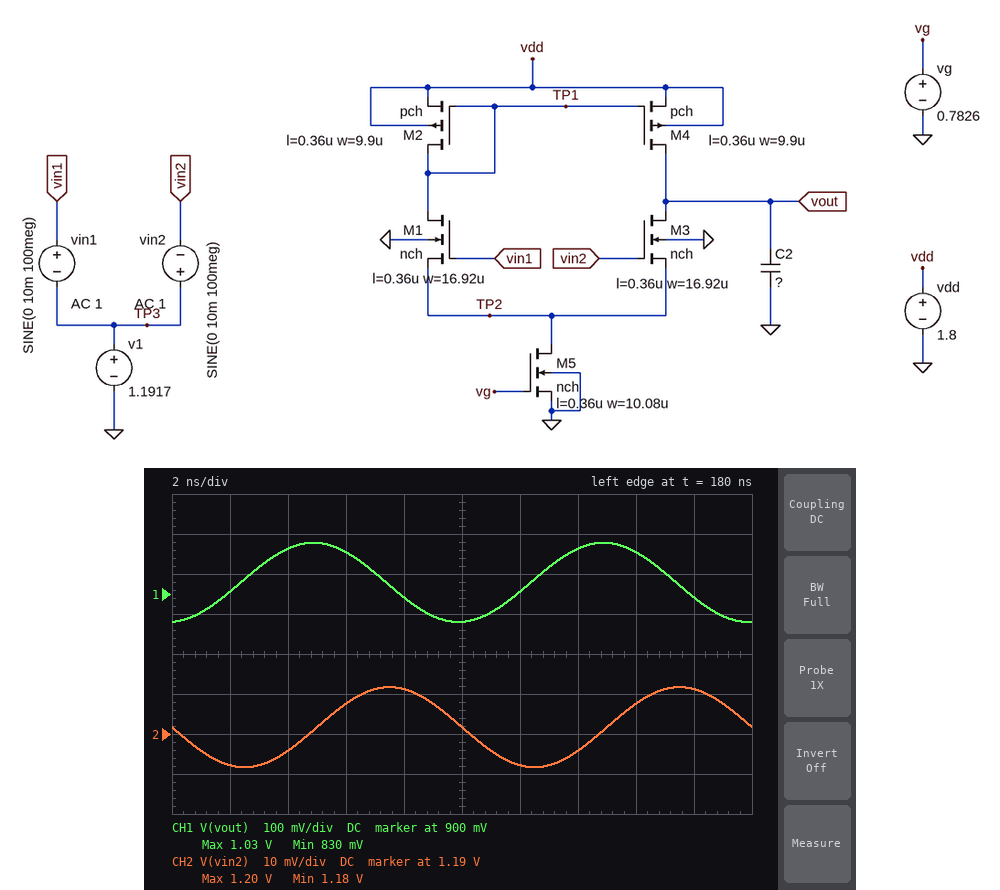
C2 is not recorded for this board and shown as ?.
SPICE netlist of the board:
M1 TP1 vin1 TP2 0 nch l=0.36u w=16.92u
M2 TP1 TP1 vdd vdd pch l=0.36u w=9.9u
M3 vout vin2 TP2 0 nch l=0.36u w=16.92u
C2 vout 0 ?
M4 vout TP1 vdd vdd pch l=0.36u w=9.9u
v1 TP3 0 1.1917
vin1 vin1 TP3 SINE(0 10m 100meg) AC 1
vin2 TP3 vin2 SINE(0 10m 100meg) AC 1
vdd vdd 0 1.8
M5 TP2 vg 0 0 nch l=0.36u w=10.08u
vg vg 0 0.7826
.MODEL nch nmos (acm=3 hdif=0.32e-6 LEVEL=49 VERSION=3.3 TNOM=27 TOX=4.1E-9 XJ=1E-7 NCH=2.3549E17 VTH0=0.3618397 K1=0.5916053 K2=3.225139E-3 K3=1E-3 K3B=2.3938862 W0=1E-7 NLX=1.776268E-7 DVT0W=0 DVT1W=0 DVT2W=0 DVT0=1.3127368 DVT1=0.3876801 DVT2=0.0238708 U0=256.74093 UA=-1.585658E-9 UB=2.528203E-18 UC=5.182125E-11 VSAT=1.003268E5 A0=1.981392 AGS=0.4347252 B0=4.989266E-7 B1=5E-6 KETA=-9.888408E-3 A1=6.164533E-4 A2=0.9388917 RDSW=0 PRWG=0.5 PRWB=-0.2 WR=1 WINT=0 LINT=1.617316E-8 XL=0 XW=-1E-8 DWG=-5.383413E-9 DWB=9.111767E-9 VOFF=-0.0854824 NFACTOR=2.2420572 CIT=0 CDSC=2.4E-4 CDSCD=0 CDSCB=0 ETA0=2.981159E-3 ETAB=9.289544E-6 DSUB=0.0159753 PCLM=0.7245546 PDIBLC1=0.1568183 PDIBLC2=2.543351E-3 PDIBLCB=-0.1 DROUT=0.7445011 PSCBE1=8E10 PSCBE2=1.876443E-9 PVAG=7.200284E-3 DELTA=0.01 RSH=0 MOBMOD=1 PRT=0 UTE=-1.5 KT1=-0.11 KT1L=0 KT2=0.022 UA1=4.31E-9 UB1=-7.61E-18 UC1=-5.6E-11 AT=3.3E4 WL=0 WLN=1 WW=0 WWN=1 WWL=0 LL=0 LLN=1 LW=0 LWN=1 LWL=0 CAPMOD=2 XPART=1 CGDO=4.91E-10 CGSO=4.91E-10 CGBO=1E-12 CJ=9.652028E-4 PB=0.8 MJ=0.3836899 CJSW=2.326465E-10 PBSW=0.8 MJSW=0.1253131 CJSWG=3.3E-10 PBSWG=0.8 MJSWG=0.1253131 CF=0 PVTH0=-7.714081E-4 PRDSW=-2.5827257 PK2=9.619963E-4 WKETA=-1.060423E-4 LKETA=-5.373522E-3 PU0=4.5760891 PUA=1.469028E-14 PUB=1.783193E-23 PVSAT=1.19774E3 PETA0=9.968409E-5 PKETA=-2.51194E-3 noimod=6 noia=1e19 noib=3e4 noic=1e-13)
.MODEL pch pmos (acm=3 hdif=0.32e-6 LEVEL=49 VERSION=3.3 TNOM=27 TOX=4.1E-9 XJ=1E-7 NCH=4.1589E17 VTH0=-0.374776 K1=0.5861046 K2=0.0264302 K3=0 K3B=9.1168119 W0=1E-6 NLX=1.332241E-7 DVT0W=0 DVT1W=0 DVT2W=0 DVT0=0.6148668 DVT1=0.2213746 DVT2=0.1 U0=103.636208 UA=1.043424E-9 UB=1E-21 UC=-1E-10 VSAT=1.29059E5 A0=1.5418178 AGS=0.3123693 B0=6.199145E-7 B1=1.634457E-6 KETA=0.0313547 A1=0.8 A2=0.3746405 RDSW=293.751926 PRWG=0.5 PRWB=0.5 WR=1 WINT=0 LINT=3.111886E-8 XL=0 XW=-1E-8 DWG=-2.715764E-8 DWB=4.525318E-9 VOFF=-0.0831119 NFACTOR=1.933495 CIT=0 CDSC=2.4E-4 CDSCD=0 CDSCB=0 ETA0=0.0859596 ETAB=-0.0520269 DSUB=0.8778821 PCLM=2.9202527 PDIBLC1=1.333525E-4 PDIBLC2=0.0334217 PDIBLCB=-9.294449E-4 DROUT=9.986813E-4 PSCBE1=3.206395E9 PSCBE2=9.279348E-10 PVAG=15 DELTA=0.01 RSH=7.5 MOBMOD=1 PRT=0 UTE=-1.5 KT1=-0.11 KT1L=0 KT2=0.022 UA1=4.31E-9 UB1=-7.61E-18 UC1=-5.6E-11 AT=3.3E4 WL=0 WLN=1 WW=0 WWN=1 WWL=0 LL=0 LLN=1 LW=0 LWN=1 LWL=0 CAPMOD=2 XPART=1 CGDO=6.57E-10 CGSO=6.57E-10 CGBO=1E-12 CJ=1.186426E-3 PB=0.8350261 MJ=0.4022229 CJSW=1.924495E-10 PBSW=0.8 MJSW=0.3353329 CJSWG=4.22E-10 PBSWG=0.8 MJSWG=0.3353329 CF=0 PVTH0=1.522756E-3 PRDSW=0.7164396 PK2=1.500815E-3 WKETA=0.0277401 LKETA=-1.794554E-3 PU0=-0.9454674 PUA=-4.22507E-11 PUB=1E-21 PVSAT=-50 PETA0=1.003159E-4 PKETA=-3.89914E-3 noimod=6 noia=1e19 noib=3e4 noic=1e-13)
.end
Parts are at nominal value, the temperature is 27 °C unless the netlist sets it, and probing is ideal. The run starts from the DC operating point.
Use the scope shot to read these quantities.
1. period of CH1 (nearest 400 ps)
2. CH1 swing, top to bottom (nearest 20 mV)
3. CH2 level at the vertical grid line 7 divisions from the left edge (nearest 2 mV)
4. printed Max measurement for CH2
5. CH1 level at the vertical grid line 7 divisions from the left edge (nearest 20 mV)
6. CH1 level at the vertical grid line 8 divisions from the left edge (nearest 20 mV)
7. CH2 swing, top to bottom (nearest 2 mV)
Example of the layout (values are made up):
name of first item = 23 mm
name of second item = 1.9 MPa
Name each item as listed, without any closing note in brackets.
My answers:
period of CH1 = 10.0 ns
CH1 swing, top to bottom = 200 mV
CH2 level at the vertical grid line 7 divisions from the left edge = 1.186 V
printed Max measurement for CH2 = 1.20 V
CH1 level at the vertical grid line 7 divisions from the left edge = 1.02 V
CH1 level at the vertical grid line 8 divisions from the left edge = 1.00 V
CH2 swing, top to bottom = 20 mV
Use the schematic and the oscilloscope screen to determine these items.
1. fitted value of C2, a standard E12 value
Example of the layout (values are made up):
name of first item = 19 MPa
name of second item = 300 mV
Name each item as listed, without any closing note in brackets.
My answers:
fitted value of C2, a standard E12 value = 560 fF
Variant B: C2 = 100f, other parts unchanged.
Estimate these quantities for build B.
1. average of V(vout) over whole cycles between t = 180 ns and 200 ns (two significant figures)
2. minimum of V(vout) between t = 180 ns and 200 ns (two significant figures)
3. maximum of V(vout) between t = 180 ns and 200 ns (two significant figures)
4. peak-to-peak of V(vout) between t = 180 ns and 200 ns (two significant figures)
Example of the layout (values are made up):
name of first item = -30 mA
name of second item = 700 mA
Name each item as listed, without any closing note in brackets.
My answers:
average of V(vout) over whole cycles between t = 180 ns and 200 ns = 960 mV
minimum of V(vout) between t = 180 ns and 200 ns = 610 mV
maximum of V(vout) between t = 180 ns and 200 ns = 1.3 V
peak-to-peak of V(vout) between t = 180 ns and 200 ns = 700 mV
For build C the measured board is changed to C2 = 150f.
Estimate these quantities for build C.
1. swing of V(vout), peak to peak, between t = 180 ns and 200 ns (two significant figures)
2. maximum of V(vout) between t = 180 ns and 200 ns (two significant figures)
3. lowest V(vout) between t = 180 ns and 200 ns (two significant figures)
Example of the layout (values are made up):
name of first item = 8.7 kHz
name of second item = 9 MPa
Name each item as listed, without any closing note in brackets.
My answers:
swing of V(vout), peak to peak, between t = 180 ns and 200 ns = 570 mV
maximum of V(vout) between t = 180 ns and 200 ns = 1.2 V
lowest V(vout) between t = 180 ns and 200 ns = 660 mV
